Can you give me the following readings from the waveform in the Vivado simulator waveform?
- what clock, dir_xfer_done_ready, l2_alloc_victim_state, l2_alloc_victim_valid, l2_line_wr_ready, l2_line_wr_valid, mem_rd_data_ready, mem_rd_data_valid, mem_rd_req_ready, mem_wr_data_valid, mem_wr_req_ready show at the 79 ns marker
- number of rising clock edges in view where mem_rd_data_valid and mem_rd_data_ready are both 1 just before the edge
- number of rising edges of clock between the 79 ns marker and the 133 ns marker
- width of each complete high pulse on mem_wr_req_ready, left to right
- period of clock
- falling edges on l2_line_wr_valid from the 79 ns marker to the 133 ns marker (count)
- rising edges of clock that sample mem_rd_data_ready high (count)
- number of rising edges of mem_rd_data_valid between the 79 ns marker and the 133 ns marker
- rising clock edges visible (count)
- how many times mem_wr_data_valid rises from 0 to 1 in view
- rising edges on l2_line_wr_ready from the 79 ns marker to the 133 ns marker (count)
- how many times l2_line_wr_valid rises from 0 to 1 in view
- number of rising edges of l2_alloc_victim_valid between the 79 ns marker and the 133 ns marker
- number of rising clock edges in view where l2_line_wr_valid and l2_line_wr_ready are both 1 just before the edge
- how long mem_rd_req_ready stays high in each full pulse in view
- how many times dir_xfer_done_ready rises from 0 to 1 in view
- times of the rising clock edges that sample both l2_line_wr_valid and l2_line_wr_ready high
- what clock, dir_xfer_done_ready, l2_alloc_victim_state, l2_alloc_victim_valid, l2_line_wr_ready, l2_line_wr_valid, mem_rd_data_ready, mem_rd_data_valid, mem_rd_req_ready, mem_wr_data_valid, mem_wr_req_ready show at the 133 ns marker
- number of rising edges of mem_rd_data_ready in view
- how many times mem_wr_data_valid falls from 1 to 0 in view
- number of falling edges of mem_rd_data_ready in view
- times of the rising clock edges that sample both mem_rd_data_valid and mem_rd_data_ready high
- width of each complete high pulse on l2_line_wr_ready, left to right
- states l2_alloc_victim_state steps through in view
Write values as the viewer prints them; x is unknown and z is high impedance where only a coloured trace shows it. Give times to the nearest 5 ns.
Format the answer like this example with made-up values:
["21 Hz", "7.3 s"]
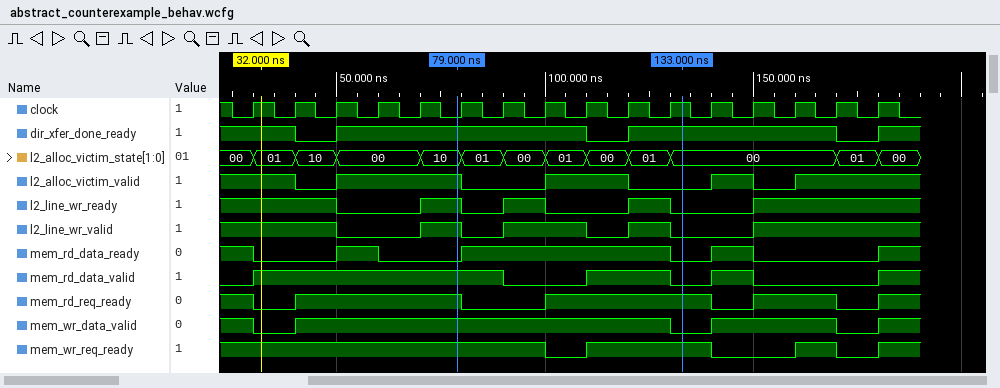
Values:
["clock=0, dir_xfer_done_ready=1, l2_alloc_victim_state=10, l2_alloc_victim_valid=1, l2_line_wr_ready=1, l2_line_wr_valid=1, mem_rd_data_ready=0, mem_rd_data_valid=1, mem_rd_req_ready=1, mem_wr_data_valid=1, mem_wr_req_ready=1", "5", "6", "30 ns, 10 ns", "10 ns", "3", "8", "1", "16", "3", "2", "4", "1", "9", "40 ns, 40 ns, 20 ns", "3", "30 ns, 40 ns, 50 ns, 80 ns, 100 ns, 130 ns, 160 ns, 170 ns, 180 ns", "clock=1, dir_xfer_done_ready=1, l2_alloc_victim_state=00, l2_alloc_victim_valid=0, l2_line_wr_ready=0, l2_line_wr_valid=0, mem_rd_data_ready=0, mem_rd_data_valid=0, mem_rd_req_ready=1, mem_wr_data_valid=0, mem_wr_req_ready=1", "4", "3", "4", "60 ns, 90 ns, 120 ns, 130 ns, 150 ns", "10 ns, 10 ns, 10 ns", "00, 01, 10, 00, 10, 01, 00, 01, 00, 01, 00, 01, 00"]
